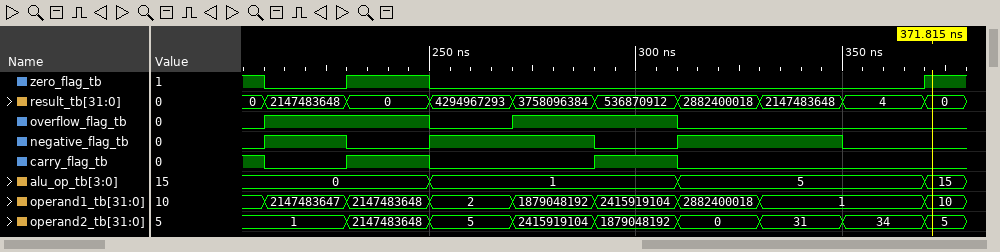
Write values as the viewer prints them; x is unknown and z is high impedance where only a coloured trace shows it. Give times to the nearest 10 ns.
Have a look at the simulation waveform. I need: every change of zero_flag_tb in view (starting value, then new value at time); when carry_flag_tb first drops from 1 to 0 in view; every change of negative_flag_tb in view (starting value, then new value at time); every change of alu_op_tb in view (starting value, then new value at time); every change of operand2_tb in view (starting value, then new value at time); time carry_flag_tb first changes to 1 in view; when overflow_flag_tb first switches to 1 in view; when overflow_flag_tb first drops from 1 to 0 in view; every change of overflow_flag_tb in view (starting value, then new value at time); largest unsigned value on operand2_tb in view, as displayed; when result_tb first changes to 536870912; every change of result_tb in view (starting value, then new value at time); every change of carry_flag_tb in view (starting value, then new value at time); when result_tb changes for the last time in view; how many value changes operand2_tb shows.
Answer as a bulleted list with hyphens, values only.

- 1, 0 at 210 ns, 1 at 230 ns, 0 at 250 ns, 1 at 370 ns
- 210 ns
- 0, 1 at 210 ns, 0 at 230 ns, 1 at 250 ns, 0 at 290 ns, 1 at 310 ns, 0 at 350 ns
- 0, 1 at 250 ns, 5 at 310 ns, 15 at 370 ns
- 1, 2147483648 at 230 ns, 5 at 250 ns, 2415919104 at 270 ns, 1879048192 at 290 ns, 0 at 310 ns, 31 at 330 ns, 34 at 350 ns, 5 at 370 ns
- 230 ns
- 210 ns
- 250 ns
- 0, 1 at 210 ns, 0 at 250 ns, 1 at 270 ns, 0 at 310 ns
- 2415919104
- 290 ns
- 0, 2147483648 at 210 ns, 0 at 230 ns, 4294967293 at 250 ns, 3758096384 at 270 ns, 536870912 at 290 ns, 2882400018 at 310 ns, 2147483648 at 330 ns, 4 at 350 ns, 0 at 370 ns
- 1, 0 at 210 ns, 1 at 230 ns, 0 at 250 ns, 1 at 290 ns, 0 at 310 ns
- 370 ns
- 8
